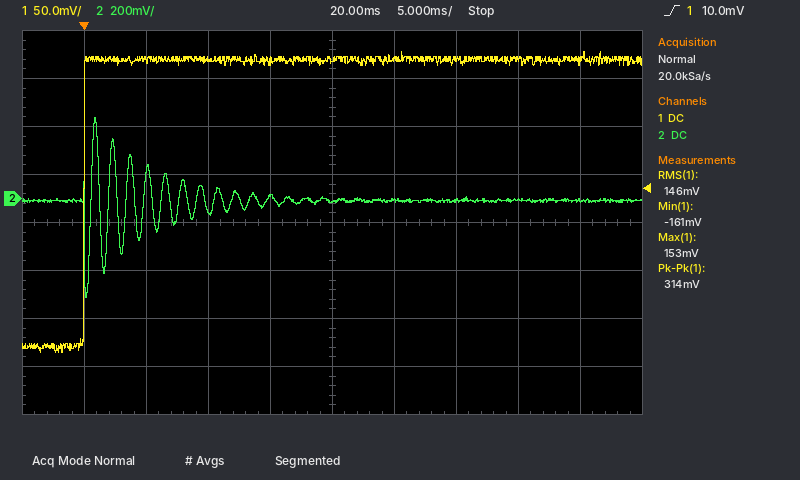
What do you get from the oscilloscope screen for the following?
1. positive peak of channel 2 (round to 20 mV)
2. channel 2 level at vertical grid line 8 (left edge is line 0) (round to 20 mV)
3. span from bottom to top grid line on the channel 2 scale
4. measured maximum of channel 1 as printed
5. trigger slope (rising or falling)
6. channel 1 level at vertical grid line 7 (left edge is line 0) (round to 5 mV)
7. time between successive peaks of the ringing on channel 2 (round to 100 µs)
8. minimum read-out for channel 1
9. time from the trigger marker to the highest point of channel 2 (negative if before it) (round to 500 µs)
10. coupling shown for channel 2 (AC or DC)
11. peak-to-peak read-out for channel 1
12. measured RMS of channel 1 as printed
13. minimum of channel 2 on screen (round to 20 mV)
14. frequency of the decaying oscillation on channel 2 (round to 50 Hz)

340 mV
0 mV
1.6 V
153 mV
rising
145 mV
1.4 ms
-161 mV
+1.0 ms
DC
314 mV
146 mV
-420 mV
700 Hz
